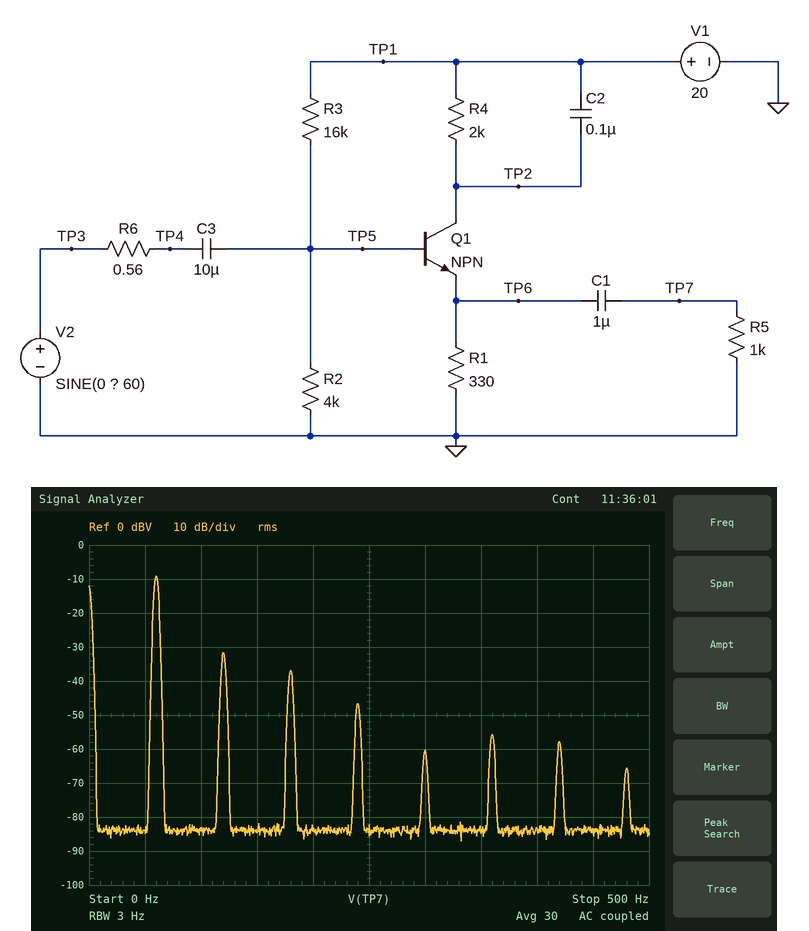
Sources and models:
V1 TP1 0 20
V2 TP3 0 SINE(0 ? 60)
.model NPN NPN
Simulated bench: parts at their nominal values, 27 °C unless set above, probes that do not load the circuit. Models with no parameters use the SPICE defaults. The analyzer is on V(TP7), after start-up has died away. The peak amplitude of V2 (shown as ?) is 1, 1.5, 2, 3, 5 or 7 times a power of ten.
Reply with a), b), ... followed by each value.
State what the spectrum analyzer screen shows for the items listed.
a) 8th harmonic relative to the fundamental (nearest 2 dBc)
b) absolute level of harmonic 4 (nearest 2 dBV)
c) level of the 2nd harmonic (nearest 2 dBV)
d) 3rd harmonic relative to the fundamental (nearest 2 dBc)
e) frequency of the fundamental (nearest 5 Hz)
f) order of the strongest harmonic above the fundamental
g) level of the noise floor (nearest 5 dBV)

a) -56 dBc
b) -46 dBV
c) -32 dBV
d) -28 dBc
e) 60 Hz
f) 2
g) -85 dBV
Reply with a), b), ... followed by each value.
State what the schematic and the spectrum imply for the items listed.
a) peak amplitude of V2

a) 1.5 V
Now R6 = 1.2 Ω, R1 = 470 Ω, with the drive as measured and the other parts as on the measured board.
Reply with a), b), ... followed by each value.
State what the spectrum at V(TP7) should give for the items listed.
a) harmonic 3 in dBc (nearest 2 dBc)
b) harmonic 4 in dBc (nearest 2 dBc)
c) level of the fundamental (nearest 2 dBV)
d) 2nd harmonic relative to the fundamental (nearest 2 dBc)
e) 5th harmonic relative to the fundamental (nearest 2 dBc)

a) -34 dBc
b) -40 dBc
c) -8 dBV
d) -30 dBc
e) -46 dBc
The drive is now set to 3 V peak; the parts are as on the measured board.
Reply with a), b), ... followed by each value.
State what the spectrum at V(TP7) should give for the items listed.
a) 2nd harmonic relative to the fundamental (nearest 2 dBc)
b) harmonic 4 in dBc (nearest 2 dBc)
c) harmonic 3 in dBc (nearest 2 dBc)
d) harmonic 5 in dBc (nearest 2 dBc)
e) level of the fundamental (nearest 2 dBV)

a) -8 dBc
b) -24 dBc
c) -14 dBc
d) -22 dBc
e) -6 dBV
